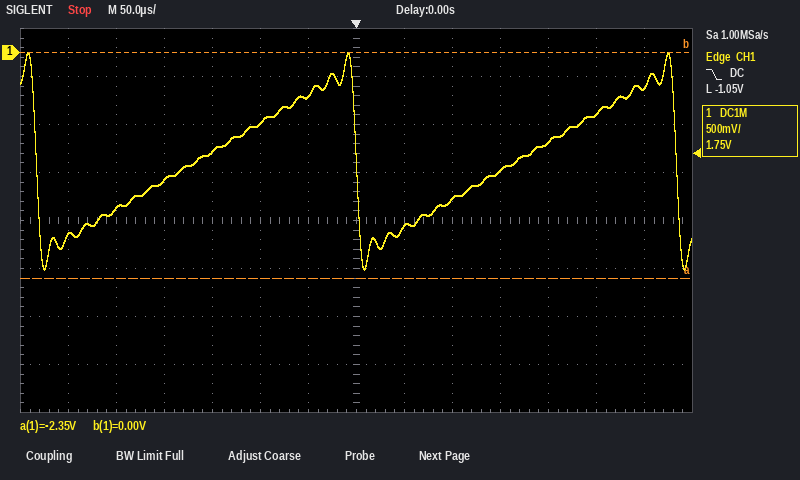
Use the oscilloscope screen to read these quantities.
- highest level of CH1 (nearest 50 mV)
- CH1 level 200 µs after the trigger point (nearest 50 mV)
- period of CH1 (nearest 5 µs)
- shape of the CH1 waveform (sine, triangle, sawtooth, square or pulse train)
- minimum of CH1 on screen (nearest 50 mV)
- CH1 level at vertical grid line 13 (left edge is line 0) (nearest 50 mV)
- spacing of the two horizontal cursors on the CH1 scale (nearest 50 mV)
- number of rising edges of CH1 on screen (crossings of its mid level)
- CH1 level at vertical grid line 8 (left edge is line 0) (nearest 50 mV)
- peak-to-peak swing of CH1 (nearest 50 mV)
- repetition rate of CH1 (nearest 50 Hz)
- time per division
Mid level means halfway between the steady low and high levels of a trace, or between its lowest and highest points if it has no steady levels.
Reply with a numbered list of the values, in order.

1. 0 mV
2. -950 mV
3. 335 µs
4. sawtooth
5. -2.25 V
6. -350 mV
7. 2.35 V
8. 2
9. -1.80 V
10. 2.25 V
11. 3.00 kHz
12. 50 µs
